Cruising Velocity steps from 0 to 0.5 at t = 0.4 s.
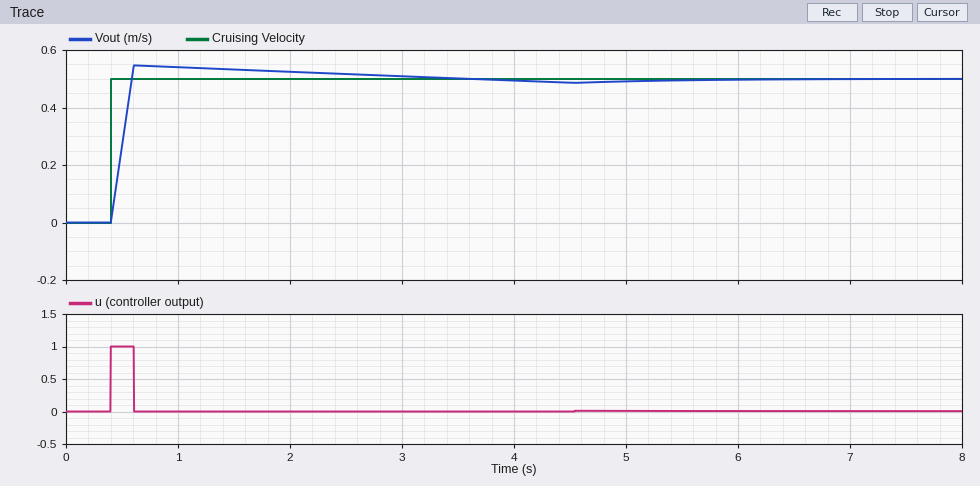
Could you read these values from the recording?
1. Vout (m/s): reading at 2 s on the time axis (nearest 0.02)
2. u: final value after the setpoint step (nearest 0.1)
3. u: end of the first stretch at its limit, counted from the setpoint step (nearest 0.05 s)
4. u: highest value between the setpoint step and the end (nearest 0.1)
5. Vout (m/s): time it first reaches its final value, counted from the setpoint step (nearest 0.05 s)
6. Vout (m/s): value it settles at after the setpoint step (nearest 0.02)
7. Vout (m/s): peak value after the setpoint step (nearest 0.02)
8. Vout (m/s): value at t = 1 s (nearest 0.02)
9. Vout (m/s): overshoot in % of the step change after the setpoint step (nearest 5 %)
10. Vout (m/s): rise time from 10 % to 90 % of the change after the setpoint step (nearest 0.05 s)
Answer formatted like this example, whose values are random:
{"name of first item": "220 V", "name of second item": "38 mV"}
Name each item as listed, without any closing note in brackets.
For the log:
{"Vout (m/s): reading at 2 s on the time axis": "0.52", "u: final value after the setpoint step": "0.0", "u: end of the first stretch at its limit, counted from the setpoint step": "0.20 s", "u: highest value between the setpoint step and the end": "1.0", "Vout (m/s): time it first reaches its final value, counted from the setpoint step": "0.20 s", "Vout (m/s): value it settles at after the setpoint step": "0.50", "Vout (m/s): peak value after the setpoint step": "0.54", "Vout (m/s): value at t = 1 s": "0.54", "Vout (m/s): overshoot in % of the step change after the setpoint step": "10 %", "Vout (m/s): rise time from 10 % to 90 % of the change after the setpoint step": "0.15 s"}
